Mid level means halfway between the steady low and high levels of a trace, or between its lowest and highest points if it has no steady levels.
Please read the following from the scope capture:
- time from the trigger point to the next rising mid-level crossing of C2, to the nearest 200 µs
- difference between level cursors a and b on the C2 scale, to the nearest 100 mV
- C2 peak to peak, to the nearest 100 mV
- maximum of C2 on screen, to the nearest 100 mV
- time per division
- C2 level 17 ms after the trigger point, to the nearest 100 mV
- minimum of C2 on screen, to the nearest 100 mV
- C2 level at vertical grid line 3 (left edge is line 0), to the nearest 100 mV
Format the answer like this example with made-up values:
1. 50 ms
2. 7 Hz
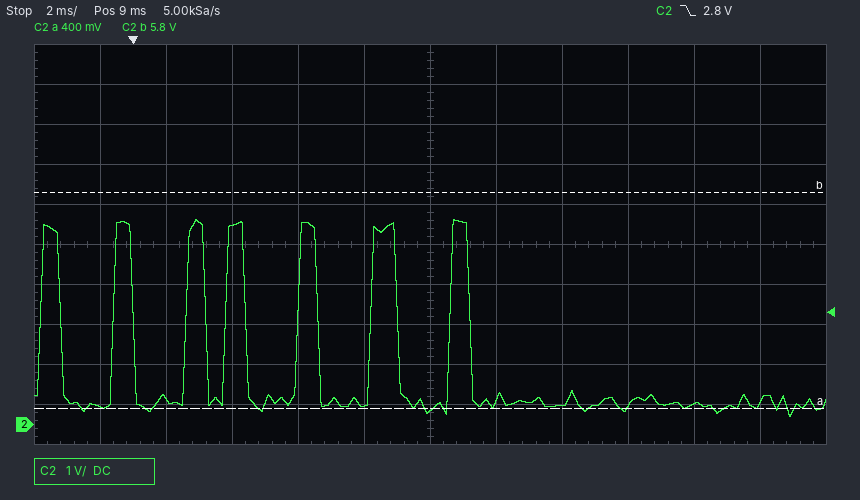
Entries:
1. 1.6 ms
2. 5.4 V
3. 4.9 V
4. 5.1 V
5. 2 ms
6. 500 mV
7. 200 mV
8. 5.0 V
